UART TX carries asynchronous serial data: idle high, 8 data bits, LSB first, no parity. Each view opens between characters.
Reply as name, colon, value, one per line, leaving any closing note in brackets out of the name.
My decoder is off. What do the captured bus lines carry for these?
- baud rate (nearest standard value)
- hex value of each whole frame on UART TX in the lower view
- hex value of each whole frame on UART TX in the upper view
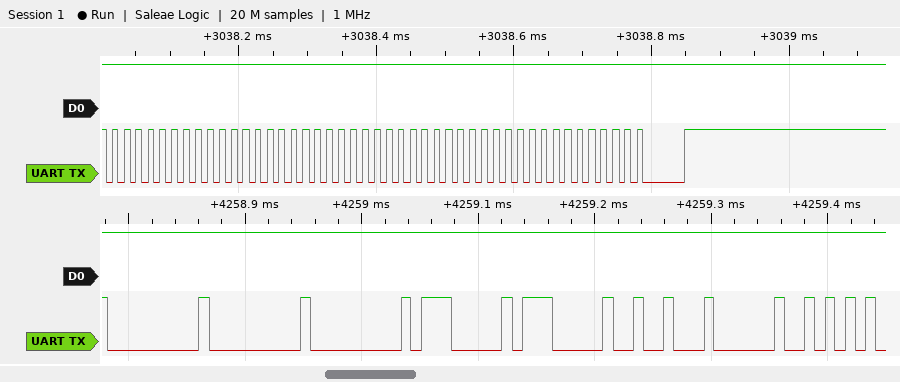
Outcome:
baud rate: 115200 baud
hex value of each whole frame on UART TX in the lower view: 00, 00, 00, 07, 07, 12, 20
hex value of each whole frame on UART TX in the upper view: 55, 55, 55, 55, 55, 55, 55, 55, 55, C0
